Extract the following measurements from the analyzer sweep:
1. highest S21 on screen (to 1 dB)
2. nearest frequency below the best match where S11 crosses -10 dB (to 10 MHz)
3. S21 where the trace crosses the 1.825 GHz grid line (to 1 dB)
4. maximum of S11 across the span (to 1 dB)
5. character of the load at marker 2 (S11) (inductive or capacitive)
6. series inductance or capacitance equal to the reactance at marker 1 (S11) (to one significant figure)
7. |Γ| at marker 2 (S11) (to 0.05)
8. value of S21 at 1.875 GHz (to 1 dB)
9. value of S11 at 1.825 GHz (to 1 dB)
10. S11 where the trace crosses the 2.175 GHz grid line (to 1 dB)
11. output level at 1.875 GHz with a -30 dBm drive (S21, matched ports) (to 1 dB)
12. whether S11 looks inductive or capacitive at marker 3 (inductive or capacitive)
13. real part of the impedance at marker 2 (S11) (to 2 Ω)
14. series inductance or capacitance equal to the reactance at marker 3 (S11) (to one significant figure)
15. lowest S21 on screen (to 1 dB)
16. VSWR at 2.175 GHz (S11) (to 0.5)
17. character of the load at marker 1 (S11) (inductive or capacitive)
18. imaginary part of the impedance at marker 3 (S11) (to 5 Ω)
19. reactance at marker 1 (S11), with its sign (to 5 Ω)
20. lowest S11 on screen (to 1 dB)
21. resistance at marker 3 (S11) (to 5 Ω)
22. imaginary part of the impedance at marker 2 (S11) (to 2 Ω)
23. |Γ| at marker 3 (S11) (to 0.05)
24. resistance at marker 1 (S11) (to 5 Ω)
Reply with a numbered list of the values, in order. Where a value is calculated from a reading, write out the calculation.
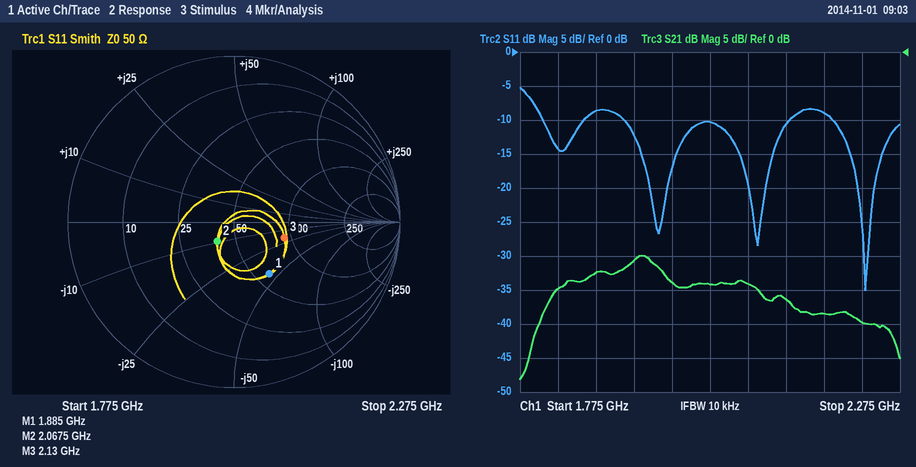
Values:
1. -30 dB
2. 2.19 GHz
3. -35 dB
4. -5 dB
5. capacitive
6. C = 1/(2π × 1.885 GHz × 45 Ω) ≈ 2 pF
7. 0.15
8. -32 dB
9. -14 dB
10. -9 dB
11. -30 dBm + (-32 dB) = -62 dBm
12. capacitive
13. 40 Ω
14. C = 1/(2π × 2.13 GHz × 20 Ω) ≈ 4 pF
15. -48 dB
16. |Γ| = 10^(-9/20) = 0.3548; VSWR = (1 + 0.3548)/(1 − 0.3548) ≈ 2.10, so 2.0 to the nearest 0.5
17. capacitive
18. -20 Ω
19. -45 Ω
20. -35 dB
21. 90 Ω
22. -10 Ω
23. 0.30
24. 60 Ω
